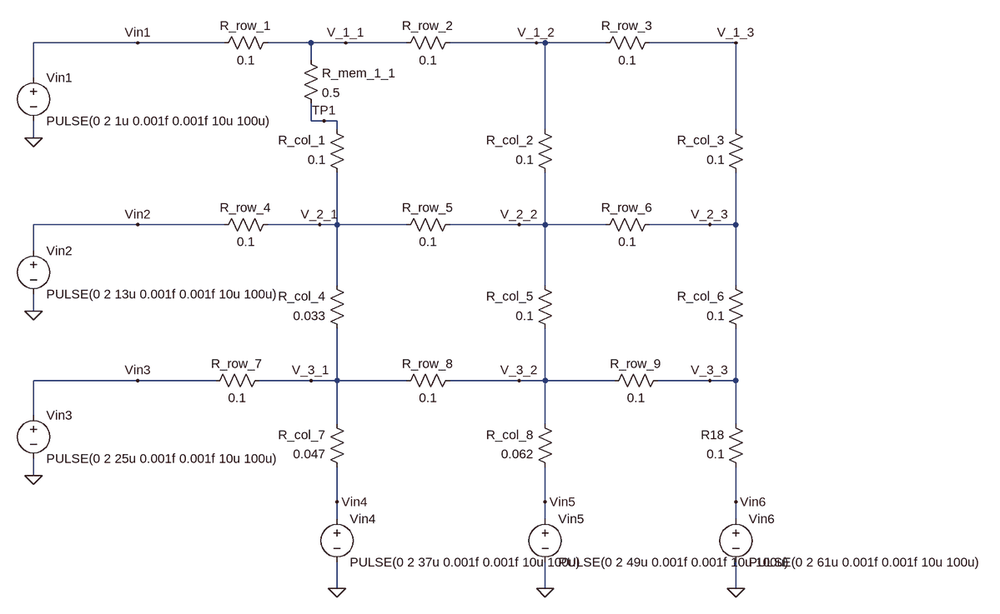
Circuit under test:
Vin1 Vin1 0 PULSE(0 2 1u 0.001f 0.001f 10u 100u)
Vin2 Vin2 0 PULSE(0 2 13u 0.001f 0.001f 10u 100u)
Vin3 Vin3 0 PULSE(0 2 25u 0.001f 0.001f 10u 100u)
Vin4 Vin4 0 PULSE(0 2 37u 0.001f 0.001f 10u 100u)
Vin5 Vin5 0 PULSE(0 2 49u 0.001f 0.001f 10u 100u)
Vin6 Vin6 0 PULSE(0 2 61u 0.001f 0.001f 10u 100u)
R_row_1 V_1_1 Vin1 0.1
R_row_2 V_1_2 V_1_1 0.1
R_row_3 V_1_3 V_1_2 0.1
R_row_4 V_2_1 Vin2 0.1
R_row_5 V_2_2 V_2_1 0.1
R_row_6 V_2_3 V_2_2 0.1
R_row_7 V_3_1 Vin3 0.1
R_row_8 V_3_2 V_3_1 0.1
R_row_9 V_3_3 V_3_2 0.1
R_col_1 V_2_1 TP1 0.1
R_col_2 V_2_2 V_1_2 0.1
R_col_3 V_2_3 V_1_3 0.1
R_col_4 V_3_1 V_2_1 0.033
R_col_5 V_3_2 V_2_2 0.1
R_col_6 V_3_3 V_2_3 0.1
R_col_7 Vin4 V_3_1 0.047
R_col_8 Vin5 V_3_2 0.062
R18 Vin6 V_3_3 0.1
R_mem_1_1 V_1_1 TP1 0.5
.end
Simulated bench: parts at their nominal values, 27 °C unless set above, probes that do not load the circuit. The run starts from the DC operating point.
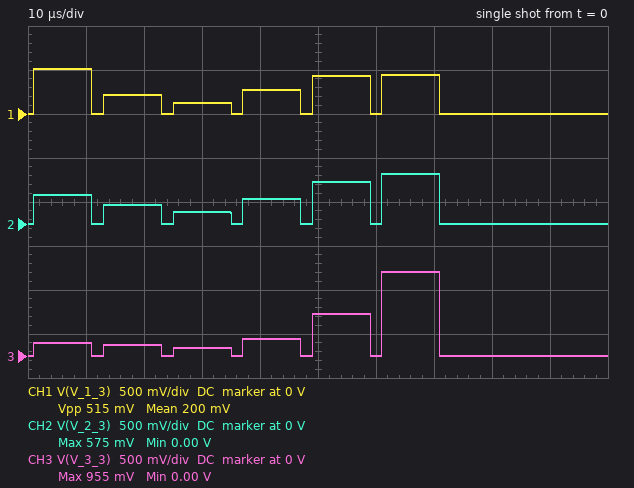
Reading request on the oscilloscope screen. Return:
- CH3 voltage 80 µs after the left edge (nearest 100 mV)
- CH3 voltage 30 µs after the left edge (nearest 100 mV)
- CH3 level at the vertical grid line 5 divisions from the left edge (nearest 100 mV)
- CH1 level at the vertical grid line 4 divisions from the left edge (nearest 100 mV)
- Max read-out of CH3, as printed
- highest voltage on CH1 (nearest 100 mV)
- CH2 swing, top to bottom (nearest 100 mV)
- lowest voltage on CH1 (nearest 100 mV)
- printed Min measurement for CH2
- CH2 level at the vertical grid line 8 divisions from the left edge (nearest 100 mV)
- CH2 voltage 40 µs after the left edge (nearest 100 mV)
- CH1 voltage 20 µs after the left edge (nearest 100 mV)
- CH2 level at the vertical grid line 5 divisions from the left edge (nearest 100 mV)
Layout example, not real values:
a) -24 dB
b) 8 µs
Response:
a) 0 V
b) 100 mV
c) 500 mV
d) 300 mV
e) 955 mV
f) 500 mV
g) 600 mV
h) 0 V
i) 0.00 V
j) 0 V
k) 300 mV
l) 200 mV
m) 500 mV
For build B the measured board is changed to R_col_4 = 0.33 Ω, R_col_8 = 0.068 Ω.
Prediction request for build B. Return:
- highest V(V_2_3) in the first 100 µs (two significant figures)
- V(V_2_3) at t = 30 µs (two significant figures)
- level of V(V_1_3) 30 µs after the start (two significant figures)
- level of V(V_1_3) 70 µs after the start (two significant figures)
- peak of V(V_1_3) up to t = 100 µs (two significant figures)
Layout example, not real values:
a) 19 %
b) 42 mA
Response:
a) 590 mV
b) 91 mV
c) 85 mV
d) 450 mV
e) 540 mV
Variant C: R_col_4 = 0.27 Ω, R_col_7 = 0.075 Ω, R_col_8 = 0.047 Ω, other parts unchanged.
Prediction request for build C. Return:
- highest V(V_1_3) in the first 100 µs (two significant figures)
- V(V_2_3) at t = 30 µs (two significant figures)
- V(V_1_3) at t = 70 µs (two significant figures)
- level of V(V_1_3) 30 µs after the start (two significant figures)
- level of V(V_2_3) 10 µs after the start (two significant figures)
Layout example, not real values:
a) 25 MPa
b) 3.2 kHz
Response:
a) 530 mV
b) 100 mV
c) 430 mV
d) 95 mV
e) 340 mV
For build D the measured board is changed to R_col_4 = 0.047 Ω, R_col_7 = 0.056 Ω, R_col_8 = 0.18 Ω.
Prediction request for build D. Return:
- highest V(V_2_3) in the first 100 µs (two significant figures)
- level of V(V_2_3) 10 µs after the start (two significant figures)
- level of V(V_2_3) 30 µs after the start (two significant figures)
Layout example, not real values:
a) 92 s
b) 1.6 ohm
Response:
a) 650 mV
b) 360 mV
c) 170 mV
